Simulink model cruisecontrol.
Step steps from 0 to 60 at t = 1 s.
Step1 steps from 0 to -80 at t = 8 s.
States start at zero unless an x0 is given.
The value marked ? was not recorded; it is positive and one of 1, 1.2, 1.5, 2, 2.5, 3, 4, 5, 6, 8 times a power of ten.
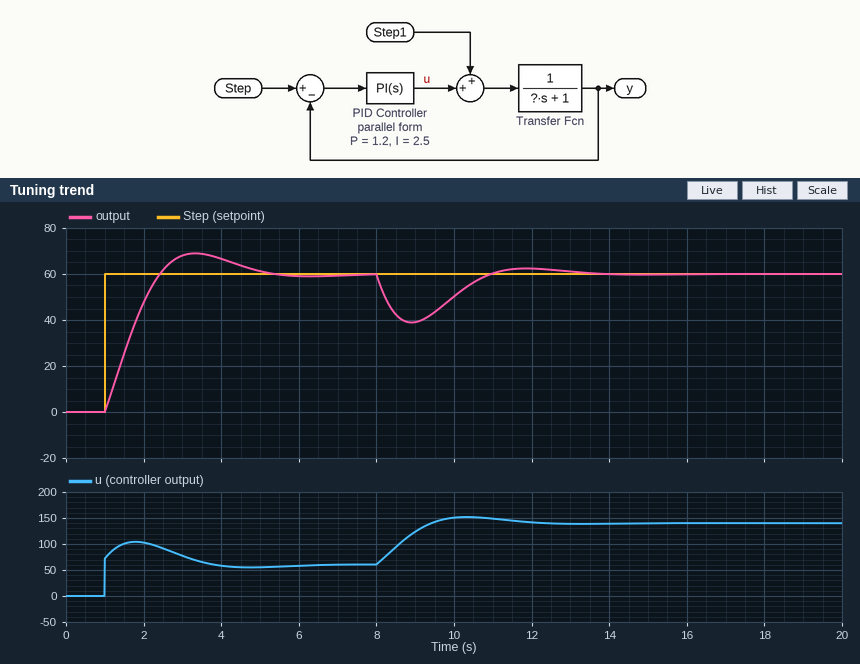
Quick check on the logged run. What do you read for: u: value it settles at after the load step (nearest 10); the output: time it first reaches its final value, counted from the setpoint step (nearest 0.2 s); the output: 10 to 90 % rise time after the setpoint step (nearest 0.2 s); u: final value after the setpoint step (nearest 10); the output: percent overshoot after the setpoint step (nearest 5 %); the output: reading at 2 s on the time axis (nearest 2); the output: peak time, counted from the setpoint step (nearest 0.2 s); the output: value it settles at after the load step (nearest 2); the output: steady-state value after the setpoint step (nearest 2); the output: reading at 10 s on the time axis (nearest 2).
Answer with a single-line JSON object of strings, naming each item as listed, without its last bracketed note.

{"u: value it settles at after the load step": "140", "the output: time it first reaches its final value, counted from the setpoint step": "1.4 s", "the output: 10 to 90 % rise time after the setpoint step": "1.0 s", "u: final value after the setpoint step": "60", "the output: percent overshoot after the setpoint step": "15 %", "the output: reading at 2 s on the time axis": "48", "the output: peak time, counted from the setpoint step": "2.4 s", "the output: value it settles at after the load step": "60", "the output: steady-state value after the setpoint step": "60", "the output: reading at 10 s on the time axis": "50"}
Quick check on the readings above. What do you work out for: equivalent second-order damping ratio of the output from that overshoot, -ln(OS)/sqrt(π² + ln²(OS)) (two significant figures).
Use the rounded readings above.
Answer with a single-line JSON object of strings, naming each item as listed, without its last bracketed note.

{"equivalent second-order damping ratio of the output from that overshoot, -ln(OS)/sqrt(π² + ln²(OS))": "0.52"}
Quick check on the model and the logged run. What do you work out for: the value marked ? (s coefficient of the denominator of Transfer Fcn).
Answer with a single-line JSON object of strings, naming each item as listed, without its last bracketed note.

{"the value marked ?": "1.5"}
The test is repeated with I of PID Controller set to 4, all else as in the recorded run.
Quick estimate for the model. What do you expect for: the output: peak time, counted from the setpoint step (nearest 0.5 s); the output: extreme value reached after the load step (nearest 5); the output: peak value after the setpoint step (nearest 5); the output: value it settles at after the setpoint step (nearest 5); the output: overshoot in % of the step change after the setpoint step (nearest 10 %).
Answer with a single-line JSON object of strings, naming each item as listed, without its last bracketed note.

{"the output: peak time, counted from the setpoint step": "2.0 s", "the output: extreme value reached after the load step": "40", "the output: peak value after the setpoint step": "75", "the output: value it settles at after the setpoint step": "60", "the output: overshoot in % of the step change after the setpoint step": "20 %"}
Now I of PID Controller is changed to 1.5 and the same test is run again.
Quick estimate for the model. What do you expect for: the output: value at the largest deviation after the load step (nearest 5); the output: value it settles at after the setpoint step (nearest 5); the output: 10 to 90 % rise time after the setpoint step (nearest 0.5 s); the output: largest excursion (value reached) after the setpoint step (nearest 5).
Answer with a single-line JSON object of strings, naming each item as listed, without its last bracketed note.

{"the output: value at the largest deviation after the load step": "35", "the output: value it settles at after the setpoint step": "60", "the output: 10 to 90 % rise time after the setpoint step": "1.5 s", "the output: largest excursion (value reached) after the setpoint step": "65"}
